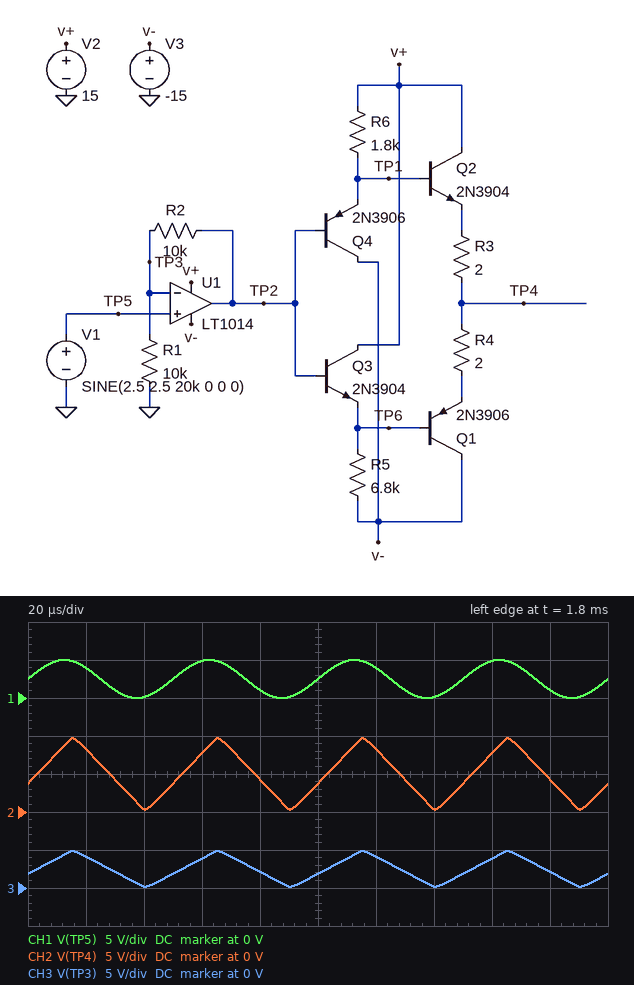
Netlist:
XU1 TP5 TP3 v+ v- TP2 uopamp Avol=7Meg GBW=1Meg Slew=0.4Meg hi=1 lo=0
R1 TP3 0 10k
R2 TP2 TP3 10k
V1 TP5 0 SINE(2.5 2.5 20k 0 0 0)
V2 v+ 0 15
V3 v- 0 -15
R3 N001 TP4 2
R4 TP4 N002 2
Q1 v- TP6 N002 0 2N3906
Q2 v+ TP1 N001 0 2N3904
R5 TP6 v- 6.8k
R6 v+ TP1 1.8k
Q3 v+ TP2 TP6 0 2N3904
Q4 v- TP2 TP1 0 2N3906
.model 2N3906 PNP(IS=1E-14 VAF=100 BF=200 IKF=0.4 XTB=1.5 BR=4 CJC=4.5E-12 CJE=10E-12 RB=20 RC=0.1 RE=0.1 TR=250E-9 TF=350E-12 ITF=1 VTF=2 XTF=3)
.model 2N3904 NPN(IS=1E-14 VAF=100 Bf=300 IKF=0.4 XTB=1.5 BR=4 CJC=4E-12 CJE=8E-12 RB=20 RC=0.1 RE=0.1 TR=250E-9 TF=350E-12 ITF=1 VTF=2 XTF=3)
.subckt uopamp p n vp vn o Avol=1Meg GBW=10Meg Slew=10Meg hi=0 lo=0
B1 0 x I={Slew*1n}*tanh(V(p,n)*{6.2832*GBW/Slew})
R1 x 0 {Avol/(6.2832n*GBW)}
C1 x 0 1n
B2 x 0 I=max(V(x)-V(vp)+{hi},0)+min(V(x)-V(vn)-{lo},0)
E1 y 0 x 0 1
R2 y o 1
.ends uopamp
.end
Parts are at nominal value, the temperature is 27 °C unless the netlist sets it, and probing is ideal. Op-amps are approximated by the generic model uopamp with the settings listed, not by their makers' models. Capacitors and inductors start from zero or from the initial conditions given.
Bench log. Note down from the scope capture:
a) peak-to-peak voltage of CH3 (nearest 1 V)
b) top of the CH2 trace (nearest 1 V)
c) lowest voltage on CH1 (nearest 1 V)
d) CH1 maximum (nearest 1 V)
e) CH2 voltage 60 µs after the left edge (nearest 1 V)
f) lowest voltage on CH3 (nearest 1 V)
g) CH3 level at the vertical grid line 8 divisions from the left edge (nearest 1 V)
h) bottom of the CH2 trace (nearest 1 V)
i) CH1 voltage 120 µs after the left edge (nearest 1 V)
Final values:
5 V
10 V
0 V
5 V
8 V
0 V
4 V
0 V
4 V
